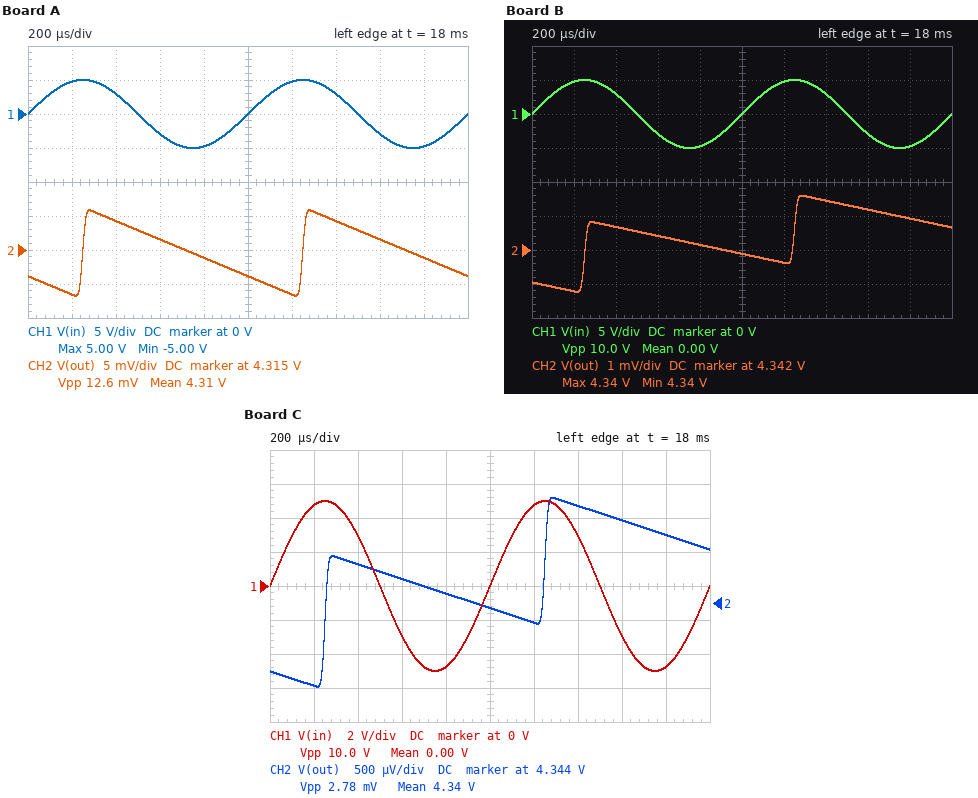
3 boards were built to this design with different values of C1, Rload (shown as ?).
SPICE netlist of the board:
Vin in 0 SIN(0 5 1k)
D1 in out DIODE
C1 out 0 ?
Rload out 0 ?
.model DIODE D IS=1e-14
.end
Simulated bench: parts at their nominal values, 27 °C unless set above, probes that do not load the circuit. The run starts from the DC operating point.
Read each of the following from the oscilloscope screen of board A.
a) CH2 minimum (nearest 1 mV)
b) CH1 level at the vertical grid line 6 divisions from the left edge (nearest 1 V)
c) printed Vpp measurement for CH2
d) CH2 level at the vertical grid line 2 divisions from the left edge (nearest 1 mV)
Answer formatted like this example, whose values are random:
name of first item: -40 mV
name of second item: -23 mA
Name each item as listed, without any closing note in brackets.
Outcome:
CH2 minimum: 4.308 V
CH1 level at the vertical grid line 6 divisions from the left edge: 5 V
printed Vpp measurement for CH2: 12.6 mV
CH2 level at the vertical grid line 2 divisions from the left edge: 4.319 V
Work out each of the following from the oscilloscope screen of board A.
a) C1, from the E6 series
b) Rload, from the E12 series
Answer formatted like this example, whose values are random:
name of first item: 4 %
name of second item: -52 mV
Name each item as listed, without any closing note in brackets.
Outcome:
C1, from the E6 series: 6.8 µF
Rload, from the E12 series: 47 kΩ
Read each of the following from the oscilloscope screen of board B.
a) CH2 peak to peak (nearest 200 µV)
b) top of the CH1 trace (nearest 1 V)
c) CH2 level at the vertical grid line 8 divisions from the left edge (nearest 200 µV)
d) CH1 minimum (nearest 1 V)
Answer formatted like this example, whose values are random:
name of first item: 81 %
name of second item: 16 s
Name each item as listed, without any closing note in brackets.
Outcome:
CH2 peak to peak: 2.8 mV
top of the CH1 trace: 5 V
CH2 level at the vertical grid line 8 divisions from the left edge: 4.3432 V
CH1 minimum: -5 V
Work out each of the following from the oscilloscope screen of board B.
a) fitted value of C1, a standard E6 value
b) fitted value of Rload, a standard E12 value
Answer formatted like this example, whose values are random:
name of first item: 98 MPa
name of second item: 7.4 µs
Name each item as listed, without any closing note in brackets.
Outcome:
fitted value of C1, a standard E6 value: 15 µF
fitted value of Rload, a standard E12 value: 220 kΩ
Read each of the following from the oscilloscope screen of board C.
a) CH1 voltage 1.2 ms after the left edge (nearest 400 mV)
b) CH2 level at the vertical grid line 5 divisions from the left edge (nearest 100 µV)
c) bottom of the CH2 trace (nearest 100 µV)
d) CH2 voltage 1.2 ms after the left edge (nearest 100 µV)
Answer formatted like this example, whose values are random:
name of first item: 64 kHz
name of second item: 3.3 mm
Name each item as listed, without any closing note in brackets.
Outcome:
CH1 voltage 1.2 ms after the left edge: 4.8 V
CH2 level at the vertical grid line 5 divisions from the left edge: 4.3439 V
bottom of the CH2 trace: 4.3428 V
CH2 voltage 1.2 ms after the left edge: 4.3437 V
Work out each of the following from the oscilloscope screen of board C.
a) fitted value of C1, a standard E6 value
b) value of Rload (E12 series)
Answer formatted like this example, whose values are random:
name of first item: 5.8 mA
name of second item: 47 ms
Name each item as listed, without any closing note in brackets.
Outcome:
fitted value of C1, a standard E6 value: 15 µF
value of Rload: 270 kΩ
